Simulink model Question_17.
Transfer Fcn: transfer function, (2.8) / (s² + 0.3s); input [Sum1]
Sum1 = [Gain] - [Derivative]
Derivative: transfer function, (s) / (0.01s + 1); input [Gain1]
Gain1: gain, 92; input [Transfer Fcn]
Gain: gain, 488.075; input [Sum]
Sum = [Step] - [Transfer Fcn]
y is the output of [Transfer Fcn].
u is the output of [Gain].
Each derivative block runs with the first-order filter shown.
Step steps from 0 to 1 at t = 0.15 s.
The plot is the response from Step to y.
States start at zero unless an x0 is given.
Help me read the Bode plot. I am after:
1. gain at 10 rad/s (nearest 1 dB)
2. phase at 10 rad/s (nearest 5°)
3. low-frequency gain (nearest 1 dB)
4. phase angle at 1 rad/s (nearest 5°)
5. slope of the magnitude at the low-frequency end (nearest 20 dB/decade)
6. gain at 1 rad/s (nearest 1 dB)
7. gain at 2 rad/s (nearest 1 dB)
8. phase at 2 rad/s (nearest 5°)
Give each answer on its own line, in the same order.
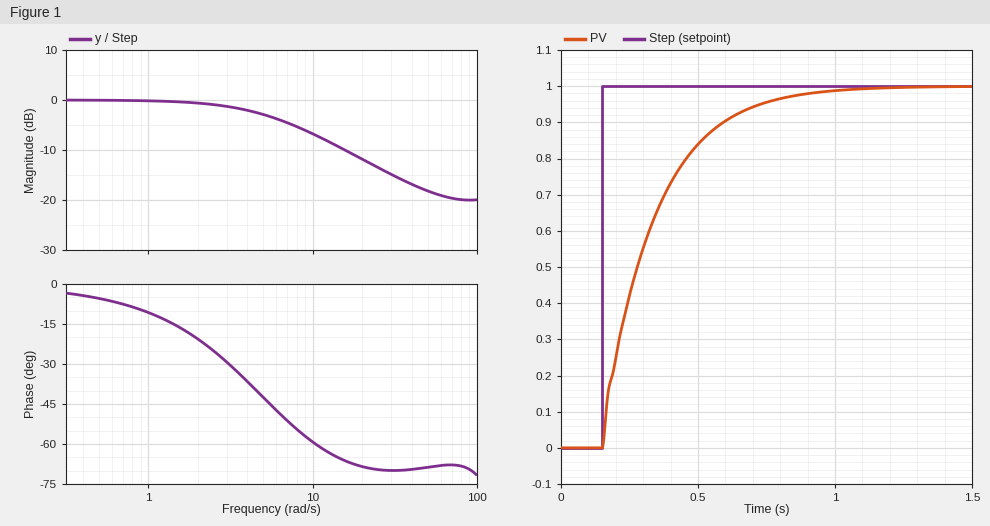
-7 dB
-60°
0 dB
-10°
0 dB/decade
0 dB
-1 dB
-20°
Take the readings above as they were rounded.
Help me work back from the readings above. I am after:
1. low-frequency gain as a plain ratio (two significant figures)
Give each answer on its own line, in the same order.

1.0
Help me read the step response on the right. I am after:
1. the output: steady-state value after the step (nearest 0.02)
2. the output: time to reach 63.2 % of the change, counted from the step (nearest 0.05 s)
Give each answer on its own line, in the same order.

1.00
0.20 s
